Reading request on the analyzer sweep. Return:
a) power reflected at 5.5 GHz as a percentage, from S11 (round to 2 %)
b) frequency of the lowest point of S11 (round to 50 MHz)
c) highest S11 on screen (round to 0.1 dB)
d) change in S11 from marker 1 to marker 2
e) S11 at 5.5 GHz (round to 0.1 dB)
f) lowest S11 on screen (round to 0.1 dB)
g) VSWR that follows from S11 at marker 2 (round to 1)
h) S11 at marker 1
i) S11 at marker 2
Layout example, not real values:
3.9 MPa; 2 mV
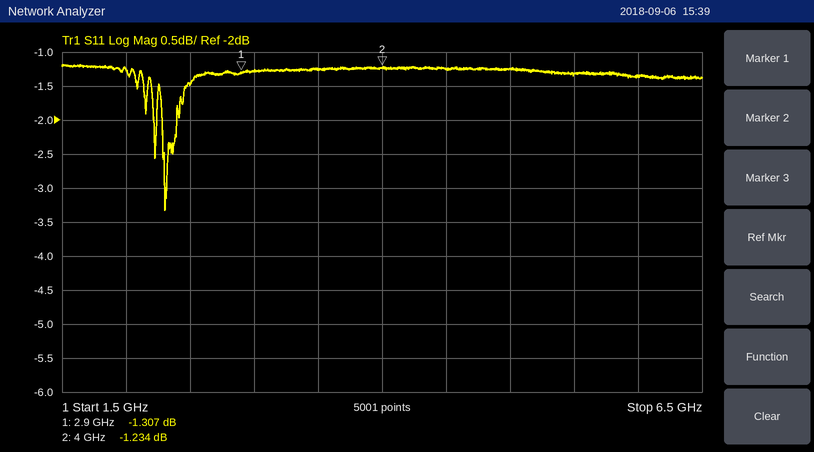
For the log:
74 %; 2.30 GHz; -1.2 dB; 0.073 dB; -1.3 dB; -3.3 dB; 14; -1.307 dB; -1.234 dB
